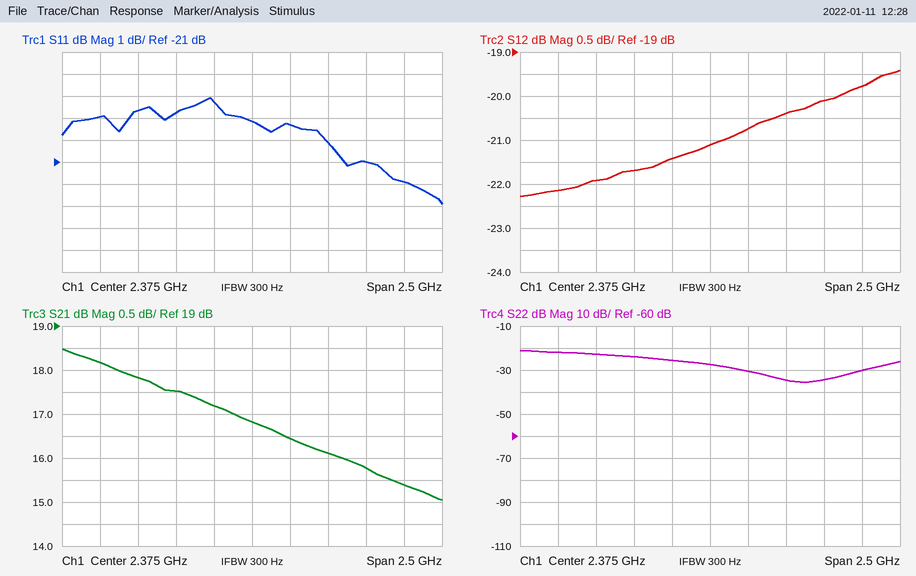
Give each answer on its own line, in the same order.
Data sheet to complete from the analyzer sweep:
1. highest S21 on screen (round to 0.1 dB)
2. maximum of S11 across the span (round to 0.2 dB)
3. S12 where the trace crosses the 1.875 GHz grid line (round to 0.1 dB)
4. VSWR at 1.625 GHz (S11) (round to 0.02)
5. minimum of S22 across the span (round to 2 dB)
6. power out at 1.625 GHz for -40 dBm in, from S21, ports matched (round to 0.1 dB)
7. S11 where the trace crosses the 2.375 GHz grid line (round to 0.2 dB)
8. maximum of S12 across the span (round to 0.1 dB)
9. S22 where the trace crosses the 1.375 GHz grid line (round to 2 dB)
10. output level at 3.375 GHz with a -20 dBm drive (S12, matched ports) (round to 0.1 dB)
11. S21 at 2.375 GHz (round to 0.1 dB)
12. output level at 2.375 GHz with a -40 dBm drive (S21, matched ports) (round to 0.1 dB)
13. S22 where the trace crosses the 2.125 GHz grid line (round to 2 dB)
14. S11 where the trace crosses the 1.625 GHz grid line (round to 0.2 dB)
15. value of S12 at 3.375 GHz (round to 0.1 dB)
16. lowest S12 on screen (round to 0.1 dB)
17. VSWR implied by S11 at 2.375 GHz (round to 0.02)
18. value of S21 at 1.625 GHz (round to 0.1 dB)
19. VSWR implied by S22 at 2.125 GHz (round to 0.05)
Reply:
18.5 dB
-18.0 dB
-21.7 dB
1.26
-36 dB
-22.2 dBm
-19.2 dB
-19.4 dB
-22 dB
-39.8 dBm
16.8 dB
-23.2 dBm
-26 dB
-18.6 dB
-19.8 dB
-22.3 dB
1.24
17.8 dB
1.10
